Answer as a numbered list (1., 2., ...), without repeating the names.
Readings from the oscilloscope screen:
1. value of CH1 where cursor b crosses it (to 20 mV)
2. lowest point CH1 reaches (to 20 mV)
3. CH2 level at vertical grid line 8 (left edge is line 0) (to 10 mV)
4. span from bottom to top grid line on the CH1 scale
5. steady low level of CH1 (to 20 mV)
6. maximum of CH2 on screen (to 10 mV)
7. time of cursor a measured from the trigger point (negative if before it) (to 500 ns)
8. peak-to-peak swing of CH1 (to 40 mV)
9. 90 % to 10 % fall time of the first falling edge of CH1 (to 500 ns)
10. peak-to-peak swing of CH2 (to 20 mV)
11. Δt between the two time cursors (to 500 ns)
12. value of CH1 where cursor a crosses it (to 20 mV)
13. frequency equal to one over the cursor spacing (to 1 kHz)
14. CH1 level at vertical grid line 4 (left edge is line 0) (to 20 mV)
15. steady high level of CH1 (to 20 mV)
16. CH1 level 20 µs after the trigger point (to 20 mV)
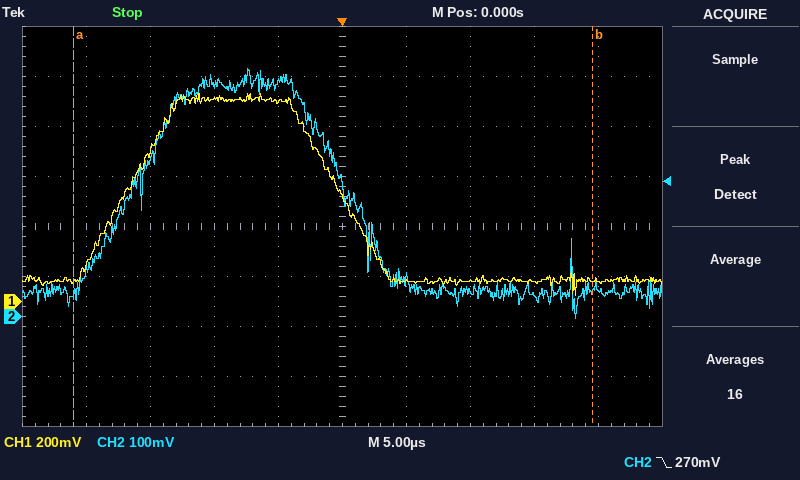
1. 80 mV
2. 20 mV
3. 40 mV
4. 1.6 V
5. 80 mV
6. 500 mV
7. -21.0 µs
8. 800 mV
9. 6.5 µs
10. 500 mV
11. 40.5 µs
12. 80 mV
13. 25 kHz
14. 800 mV
15. 800 mV
16. 80 mV
